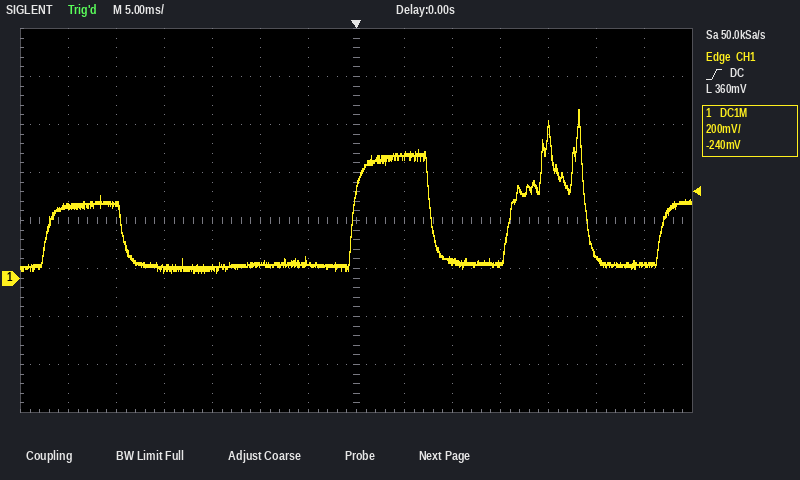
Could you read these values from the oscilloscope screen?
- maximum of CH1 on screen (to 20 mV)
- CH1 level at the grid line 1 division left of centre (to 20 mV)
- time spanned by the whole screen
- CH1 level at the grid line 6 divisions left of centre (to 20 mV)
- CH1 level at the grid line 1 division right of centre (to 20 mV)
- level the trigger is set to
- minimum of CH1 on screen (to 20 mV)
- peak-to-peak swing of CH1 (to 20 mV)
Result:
700 mV
60 mV
70 ms
300 mV
520 mV
360 mV
20 mV
680 mV
